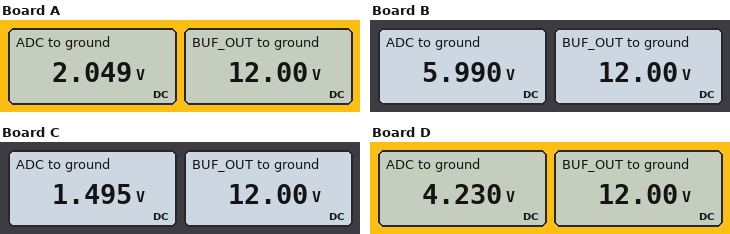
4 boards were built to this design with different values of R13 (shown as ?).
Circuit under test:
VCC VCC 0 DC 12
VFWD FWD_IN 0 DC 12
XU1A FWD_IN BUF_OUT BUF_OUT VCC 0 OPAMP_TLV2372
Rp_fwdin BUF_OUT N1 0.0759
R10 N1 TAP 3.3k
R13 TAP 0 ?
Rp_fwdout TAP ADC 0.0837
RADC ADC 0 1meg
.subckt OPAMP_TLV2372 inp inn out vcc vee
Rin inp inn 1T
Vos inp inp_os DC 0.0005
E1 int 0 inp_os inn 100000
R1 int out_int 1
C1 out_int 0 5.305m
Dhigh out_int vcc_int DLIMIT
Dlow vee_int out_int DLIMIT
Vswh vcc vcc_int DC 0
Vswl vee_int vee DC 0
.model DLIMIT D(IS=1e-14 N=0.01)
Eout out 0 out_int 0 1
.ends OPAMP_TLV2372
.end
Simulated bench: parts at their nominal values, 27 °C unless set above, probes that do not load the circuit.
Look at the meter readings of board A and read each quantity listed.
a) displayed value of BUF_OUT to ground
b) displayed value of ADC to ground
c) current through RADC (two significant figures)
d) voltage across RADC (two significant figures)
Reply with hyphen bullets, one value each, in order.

- 12.00 V
- 2.049 V
- 2.0 µA
- 2.0 V
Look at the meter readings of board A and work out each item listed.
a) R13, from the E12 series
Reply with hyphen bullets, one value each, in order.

- 680 Ω
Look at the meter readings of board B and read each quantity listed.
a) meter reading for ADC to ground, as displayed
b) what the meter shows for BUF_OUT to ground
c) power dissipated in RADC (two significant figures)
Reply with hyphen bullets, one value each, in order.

- 5.990 V
- 12.00 V
- 36 µW
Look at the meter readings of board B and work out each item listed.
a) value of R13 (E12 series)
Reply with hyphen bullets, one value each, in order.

- 3.3 kΩ
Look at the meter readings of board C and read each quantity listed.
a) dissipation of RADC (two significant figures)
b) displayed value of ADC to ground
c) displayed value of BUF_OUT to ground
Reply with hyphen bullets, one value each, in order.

- 2.2 µW
- 1.495 V
- 12.00 V
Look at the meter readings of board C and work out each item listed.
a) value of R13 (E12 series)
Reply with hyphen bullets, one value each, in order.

- 470 Ω
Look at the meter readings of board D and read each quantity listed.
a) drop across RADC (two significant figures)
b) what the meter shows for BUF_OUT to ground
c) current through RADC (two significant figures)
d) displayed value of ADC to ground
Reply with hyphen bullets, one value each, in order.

- 4.2 V
- 12.00 V
- 4.2 µA
- 4.230 V
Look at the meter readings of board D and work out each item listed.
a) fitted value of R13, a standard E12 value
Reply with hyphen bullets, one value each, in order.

- 1.8 kΩ
